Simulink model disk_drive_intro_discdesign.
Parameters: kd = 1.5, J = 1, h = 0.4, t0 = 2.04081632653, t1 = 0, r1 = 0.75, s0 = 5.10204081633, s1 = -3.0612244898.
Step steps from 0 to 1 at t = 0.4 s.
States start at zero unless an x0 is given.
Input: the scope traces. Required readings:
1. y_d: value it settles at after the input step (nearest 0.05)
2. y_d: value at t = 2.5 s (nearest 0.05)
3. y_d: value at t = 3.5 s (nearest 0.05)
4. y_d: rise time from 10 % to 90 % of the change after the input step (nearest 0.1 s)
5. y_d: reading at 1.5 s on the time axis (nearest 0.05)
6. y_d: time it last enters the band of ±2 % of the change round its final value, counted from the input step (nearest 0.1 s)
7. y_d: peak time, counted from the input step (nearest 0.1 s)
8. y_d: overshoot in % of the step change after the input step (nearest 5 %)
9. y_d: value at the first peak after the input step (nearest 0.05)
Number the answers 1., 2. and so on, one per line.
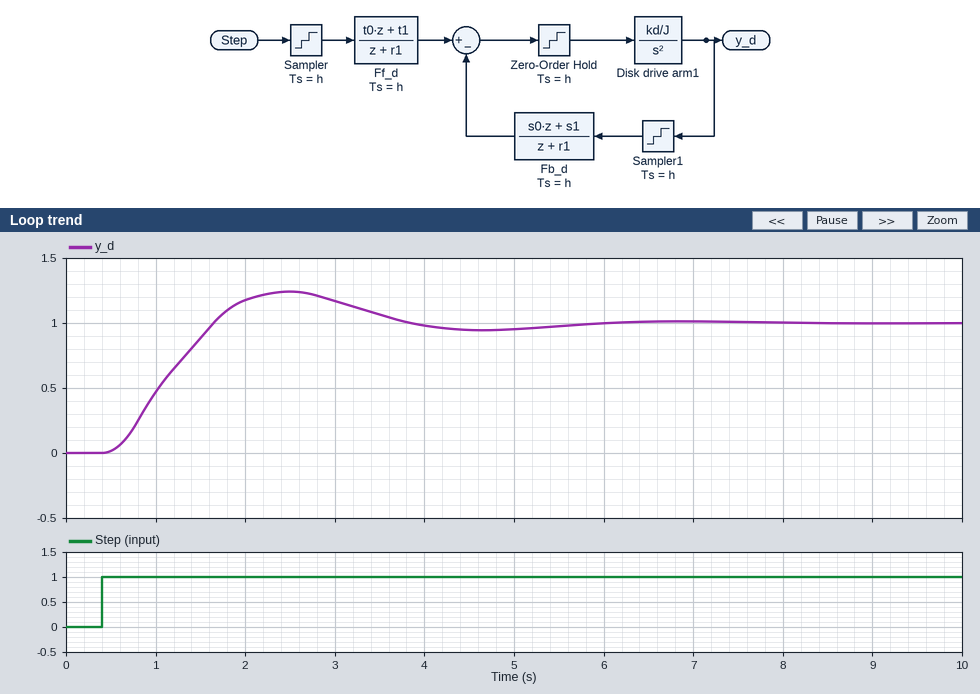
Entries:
1. 1.00
2. 1.25
3. 1.05
4. 0.9 s
5. 0.90
6. 5.2 s
7. 2.1 s
8. 25 %
9. 1.25
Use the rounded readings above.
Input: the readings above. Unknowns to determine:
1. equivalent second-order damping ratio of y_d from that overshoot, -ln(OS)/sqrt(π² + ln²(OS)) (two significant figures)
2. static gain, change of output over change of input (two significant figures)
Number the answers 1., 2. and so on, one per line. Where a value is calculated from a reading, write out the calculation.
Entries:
1. ln(0.25) = -1.386; 1.386 / sqrt(9.870 + 1.922) = 0.40
2. (1 - 0) / (1 - 0) = 1.0
